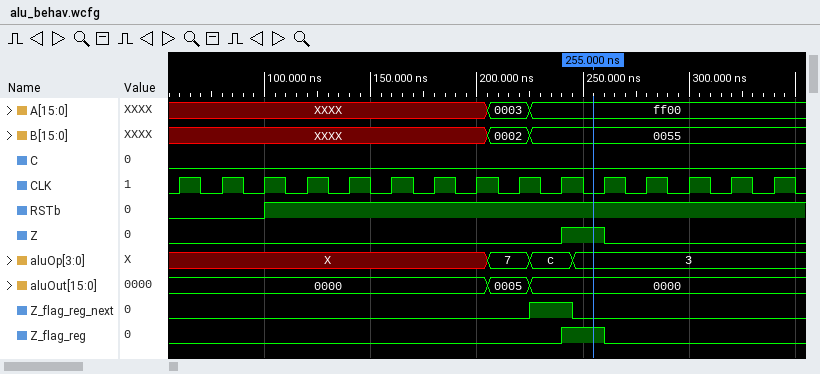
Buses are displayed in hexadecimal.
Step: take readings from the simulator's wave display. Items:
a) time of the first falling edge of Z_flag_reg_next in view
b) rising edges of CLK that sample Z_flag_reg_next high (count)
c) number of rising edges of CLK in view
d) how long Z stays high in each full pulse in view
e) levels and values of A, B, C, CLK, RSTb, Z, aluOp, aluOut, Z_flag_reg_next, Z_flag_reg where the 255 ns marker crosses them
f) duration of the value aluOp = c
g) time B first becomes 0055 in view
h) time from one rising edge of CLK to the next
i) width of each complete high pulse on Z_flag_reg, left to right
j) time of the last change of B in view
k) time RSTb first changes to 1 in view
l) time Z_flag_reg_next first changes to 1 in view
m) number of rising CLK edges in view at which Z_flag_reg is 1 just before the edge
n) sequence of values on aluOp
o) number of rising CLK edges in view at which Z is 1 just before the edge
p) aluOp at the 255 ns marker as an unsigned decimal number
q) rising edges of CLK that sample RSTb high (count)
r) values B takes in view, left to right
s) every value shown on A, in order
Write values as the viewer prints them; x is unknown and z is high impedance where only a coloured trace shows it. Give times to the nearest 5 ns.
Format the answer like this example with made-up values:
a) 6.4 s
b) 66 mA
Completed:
a) 245 ns
b) 1
c) 15
d) 20 ns
e) A=ff00, B=0055, C=0, CLK=0, RSTb=1, Z=1, aluOp=3, aluOut=0000, Z_flag_reg_next=0, Z_flag_reg=1
f) 20 ns
g) 225 ns
h) 20 ns
i) 20 ns
j) 225 ns
k) 100 ns
l) 225 ns
m) 1
n) X, 7, c, 3
o) 1
p) 3
q) 12
r) XXXX, 0002, 0055
s) XXXX, 0003, ff00
